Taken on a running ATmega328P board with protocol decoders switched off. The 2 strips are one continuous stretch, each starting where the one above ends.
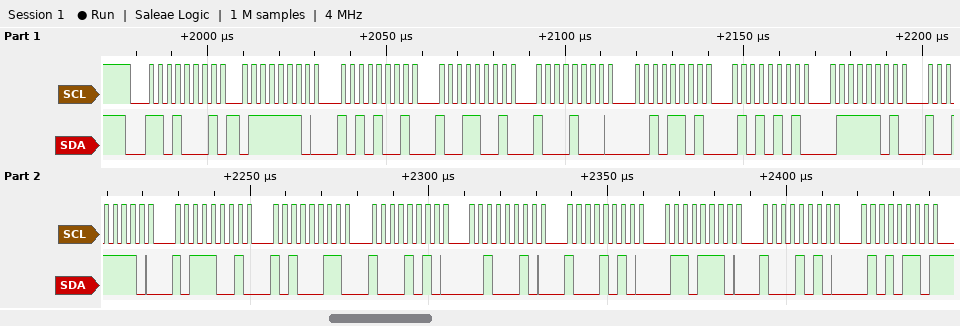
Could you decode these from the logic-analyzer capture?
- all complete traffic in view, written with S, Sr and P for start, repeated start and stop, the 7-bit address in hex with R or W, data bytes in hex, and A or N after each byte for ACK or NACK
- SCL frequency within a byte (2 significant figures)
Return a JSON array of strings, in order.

["S 68R A 7E A A9 A 99 A 88 A 2D A 55 A 7D A 9E A B9 A A3 A 8A A 22 A 8A A 6E A 8A A 56 N", "400 kHz"]
